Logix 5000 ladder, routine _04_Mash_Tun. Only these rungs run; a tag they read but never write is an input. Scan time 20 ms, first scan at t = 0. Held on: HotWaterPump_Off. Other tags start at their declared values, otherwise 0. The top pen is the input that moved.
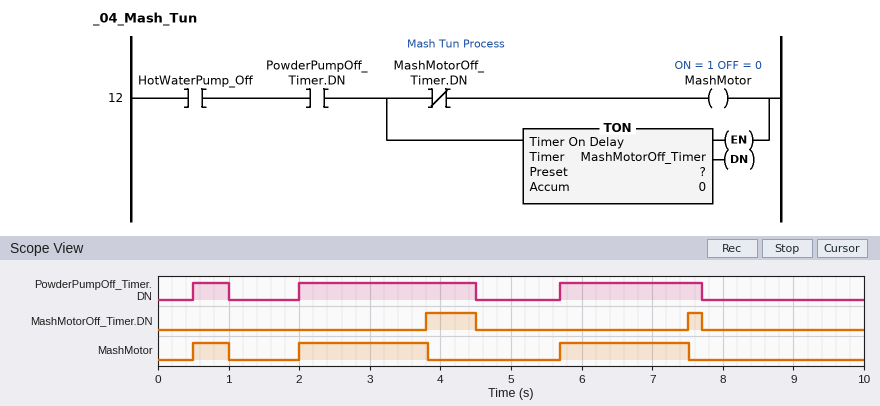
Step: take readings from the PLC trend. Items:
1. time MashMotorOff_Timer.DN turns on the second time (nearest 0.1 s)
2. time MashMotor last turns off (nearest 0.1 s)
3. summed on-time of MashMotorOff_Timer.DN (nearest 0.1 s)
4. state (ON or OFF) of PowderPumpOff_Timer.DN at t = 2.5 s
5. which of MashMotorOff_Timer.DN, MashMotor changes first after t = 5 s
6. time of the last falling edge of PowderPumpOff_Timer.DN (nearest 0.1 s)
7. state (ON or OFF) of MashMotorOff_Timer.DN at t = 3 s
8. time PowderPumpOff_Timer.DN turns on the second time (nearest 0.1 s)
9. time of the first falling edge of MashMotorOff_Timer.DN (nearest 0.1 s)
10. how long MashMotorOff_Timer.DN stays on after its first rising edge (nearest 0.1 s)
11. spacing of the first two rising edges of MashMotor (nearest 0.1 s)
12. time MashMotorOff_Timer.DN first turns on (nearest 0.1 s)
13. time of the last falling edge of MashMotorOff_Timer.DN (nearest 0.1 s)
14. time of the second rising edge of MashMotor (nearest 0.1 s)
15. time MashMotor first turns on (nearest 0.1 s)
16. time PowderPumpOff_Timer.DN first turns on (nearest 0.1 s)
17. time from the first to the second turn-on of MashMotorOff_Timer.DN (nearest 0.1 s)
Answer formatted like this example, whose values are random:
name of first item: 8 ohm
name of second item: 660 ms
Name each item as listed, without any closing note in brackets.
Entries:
time MashMotorOff_Timer.DN turns on the second time: 7.5 s
time MashMotor last turns off: 7.5 s
summed on-time of MashMotorOff_Timer.DN: 0.9 s
state (ON or OFF) of PowderPumpOff_Timer.DN at t = 2.5 s: ON
which of MashMotorOff_Timer.DN, MashMotor changes first after t = 5 s: MashMotor
time of the last falling edge of PowderPumpOff_Timer.DN: 7.7 s
state (ON or OFF) of MashMotorOff_Timer.DN at t = 3 s: OFF
time PowderPumpOff_Timer.DN turns on the second time: 2.0 s
time of the first falling edge of MashMotorOff_Timer.DN: 4.5 s
how long MashMotorOff_Timer.DN stays on after its first rising edge: 0.7 s
spacing of the first two rising edges of MashMotor: 1.5 s
time MashMotorOff_Timer.DN first turns on: 3.8 s
time of the last falling edge of MashMotorOff_Timer.DN: 7.7 s
time of the second rising edge of MashMotor: 2.0 s
time MashMotor first turns on: 0.5 s
time PowderPumpOff_Timer.DN first turns on: 0.5 s
time from the first to the second turn-on of MashMotorOff_Timer.DN: 3.7 s
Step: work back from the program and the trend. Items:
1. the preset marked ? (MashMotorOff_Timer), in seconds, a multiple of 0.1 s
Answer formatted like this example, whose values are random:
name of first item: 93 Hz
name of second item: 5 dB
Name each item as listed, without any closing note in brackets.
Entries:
the preset marked ? (MashMotorOff_Timer), in seconds, a multiple of 0.1 s: 1.8 s
